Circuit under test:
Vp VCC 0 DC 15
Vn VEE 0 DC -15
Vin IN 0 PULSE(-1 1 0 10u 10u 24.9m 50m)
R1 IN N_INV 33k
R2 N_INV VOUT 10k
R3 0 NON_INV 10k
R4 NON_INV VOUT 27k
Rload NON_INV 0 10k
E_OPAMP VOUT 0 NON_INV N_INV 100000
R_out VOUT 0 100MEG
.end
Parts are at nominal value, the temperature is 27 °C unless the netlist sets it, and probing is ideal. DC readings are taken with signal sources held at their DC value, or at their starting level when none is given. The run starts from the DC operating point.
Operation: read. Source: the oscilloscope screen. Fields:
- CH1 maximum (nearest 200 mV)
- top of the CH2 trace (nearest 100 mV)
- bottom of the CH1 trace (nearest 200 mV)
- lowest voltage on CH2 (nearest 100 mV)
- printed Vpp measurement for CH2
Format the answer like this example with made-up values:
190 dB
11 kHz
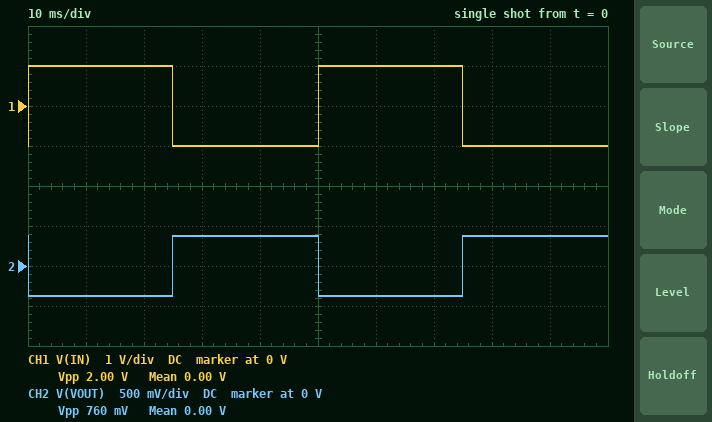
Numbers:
1.0 V
400 mV
-1.0 V
-400 mV
760 mV
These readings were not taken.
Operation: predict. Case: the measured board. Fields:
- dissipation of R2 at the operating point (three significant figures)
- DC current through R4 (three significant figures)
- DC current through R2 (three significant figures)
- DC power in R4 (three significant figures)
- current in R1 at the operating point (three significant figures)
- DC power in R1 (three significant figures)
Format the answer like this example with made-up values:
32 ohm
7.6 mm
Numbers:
10.3 µW
11.9 µA
32.1 µA
3.82 µW
32.1 µA
34.0 µW
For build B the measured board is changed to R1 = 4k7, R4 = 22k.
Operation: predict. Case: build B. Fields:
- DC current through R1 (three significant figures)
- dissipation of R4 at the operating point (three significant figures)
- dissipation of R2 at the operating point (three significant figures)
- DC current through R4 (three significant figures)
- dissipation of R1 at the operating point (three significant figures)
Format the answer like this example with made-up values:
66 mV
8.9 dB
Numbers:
412 µA
771 µW
1.70 mW
187 µA
798 µW
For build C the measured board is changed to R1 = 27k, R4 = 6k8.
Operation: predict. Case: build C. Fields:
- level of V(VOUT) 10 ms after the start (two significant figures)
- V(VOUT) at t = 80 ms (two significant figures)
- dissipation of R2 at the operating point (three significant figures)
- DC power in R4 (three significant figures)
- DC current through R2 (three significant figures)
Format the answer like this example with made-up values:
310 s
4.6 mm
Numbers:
-880 mV
880 mV
25.9 µW
38.1 µW
50.9 µA
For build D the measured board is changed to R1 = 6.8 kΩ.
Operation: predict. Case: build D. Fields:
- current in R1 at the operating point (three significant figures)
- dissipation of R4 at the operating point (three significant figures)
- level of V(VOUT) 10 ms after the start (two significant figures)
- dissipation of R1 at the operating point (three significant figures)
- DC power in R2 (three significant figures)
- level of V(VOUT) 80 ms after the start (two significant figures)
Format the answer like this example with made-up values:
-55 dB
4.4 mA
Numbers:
202 µA
151 µW
-2.4 V
278 µW
408 µW
2.4 V
